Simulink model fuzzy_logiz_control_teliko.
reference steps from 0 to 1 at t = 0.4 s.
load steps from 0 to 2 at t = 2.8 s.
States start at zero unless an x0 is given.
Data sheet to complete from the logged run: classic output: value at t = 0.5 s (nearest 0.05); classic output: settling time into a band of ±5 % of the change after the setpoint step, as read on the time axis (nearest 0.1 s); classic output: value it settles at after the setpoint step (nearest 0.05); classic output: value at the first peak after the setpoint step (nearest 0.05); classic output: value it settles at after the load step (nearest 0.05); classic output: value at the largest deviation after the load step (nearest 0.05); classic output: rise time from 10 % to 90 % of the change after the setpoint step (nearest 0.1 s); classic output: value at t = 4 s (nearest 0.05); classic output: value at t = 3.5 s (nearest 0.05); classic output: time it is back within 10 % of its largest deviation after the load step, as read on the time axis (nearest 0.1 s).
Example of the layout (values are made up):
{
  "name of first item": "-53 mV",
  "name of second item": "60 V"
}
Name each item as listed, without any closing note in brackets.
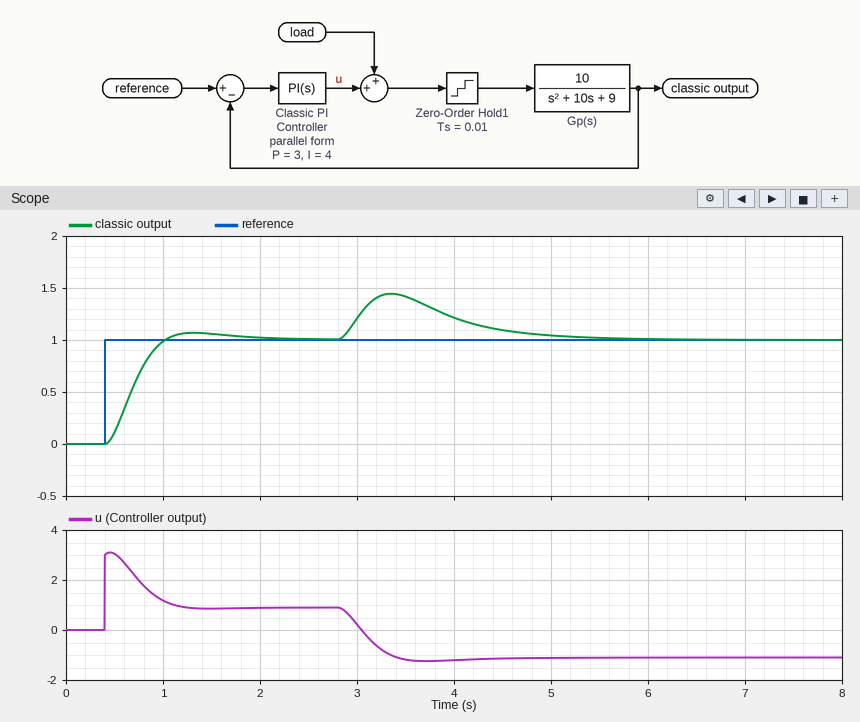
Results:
{
  "classic output: value at t = 0.5 s": "0.10",
  "classic output: settling time into a band of ±5 % of the change after the setpoint step, as read on the time axis": "1.6 s",
  "classic output: value it settles at after the setpoint step": "1.00",
  "classic output: value at the first peak after the setpoint step": "1.05",
  "classic output: value it settles at after the load step": "1.00",
  "classic output: value at the largest deviation after the load step": "1.45",
  "classic output: rise time from 10 % to 90 % of the change after the setpoint step": "0.4 s",
  "classic output: value at t = 4 s": "1.20",
  "classic output: value at t = 3.5 s": "1.40",
  "classic output: time it is back within 10 % of its largest deviation after the load step, as read on the time axis": "5.0 s"
}
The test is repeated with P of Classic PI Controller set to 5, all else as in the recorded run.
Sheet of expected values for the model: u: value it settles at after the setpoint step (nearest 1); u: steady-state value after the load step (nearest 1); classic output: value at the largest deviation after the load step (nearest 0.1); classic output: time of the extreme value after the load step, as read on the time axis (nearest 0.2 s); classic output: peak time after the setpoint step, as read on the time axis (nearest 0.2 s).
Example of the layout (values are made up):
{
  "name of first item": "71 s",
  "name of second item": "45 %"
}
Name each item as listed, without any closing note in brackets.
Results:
{
  "u: value it settles at after the setpoint step": "1",
  "u: steady-state value after the load step": "-1",
  "classic output: value at the largest deviation after the load step": "1.3",
  "classic output: time of the extreme value after the load step, as read on the time axis": "3.2 s",
  "classic output: peak time after the setpoint step, as read on the time axis": "1.0 s"
}
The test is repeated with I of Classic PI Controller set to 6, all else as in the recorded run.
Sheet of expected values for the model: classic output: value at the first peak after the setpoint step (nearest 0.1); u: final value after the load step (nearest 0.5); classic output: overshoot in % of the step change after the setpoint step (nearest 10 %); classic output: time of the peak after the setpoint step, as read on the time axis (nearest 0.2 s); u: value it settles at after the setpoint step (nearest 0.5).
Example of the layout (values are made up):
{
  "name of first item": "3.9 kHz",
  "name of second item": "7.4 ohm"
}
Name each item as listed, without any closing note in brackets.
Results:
{
  "classic output: value at the first peak after the setpoint step": "1.2",
  "u: final value after the load step": "-1.0",
  "classic output: overshoot in % of the step change after the setpoint step": "20 %",
  "classic output: time of the peak after the setpoint step, as read on the time axis": "1.2 s",
  "u: value it settles at after the setpoint step": "1.0"
}
